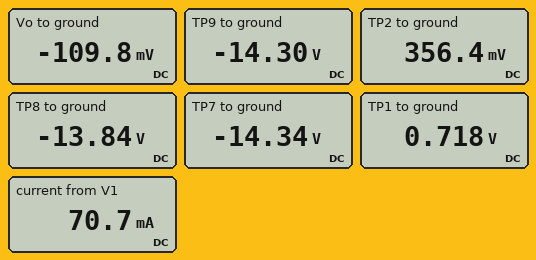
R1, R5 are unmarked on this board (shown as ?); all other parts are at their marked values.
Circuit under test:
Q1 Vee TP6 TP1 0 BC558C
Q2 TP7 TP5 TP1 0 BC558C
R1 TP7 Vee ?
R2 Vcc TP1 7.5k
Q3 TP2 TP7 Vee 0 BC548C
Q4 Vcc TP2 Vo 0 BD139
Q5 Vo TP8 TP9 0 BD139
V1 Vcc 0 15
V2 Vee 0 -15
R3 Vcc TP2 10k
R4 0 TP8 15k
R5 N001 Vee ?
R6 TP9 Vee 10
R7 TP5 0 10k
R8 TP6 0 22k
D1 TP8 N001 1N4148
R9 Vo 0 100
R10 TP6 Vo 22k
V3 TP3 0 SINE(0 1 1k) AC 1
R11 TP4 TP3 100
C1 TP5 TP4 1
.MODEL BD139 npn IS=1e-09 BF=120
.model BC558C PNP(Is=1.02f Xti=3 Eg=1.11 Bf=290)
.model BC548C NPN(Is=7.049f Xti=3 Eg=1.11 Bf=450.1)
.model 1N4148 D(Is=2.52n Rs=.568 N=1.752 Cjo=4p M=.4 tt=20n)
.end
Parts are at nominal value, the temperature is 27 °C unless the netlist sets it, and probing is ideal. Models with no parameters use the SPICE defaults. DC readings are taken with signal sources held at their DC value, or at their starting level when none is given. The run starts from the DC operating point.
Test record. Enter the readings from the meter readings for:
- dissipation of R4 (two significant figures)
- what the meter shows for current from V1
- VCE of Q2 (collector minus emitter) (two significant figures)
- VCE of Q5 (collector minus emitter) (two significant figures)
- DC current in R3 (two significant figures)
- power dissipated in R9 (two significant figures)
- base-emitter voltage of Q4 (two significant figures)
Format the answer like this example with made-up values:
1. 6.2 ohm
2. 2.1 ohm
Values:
1. 13 mW
2. 70.7 mA
3. -15 V
4. 14 V
5. 1.5 mA
6. 120 µW
7. 470 mV
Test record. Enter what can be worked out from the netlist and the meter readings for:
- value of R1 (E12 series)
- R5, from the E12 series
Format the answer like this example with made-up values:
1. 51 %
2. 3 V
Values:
1. 1.2 kΩ
2. 1.8 kΩ
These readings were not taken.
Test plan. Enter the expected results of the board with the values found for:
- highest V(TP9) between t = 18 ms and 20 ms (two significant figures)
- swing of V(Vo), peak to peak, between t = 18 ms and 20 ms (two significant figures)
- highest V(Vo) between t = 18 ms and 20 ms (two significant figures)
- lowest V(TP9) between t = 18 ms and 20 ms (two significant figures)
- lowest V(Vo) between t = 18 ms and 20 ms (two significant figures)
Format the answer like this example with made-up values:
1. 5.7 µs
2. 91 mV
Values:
1. -14 V
2. 4.0 V
3. 1.9 V
4. -14 V
5. -2.1 V
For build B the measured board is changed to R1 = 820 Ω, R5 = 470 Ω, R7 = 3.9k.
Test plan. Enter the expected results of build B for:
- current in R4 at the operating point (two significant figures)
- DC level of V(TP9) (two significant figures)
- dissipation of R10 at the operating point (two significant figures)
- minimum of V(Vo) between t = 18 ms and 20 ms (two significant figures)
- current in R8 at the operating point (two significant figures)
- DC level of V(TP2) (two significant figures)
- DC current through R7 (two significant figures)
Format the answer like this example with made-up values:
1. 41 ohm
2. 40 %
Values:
1. 940 µA
2. -15 V
3. 280 nW
4. -2.0 V
5. 170 nA
6. 380 mV
7. 2.8 µA
